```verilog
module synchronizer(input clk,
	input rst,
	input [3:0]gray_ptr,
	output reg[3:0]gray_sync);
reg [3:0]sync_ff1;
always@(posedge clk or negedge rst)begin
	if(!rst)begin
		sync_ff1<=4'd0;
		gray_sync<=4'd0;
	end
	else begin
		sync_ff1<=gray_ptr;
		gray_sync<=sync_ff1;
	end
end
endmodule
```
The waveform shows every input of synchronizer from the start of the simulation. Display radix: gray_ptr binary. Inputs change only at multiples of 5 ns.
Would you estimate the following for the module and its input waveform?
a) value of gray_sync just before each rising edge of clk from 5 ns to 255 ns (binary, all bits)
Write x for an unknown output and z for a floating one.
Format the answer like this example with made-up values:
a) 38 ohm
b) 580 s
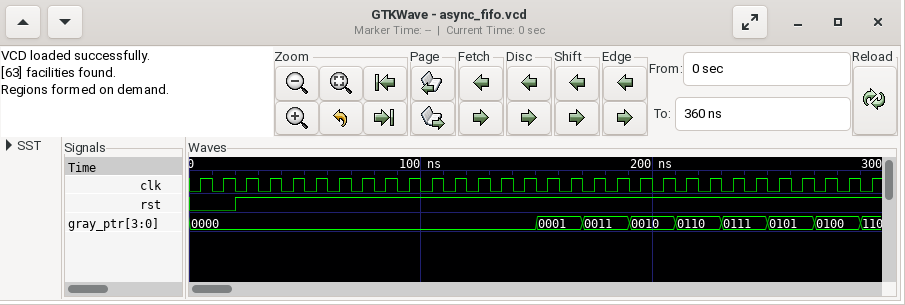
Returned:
a) 0000, 0000, 0000, 0000, 0000, 0000, 0000, 0000, 0000, 0000, 0000, 0000, 0000, 0000, 0000, 0000, 0000, 0001, 0001, 0011, 0011, 0010, 0010, 0110, 0110, 0111
